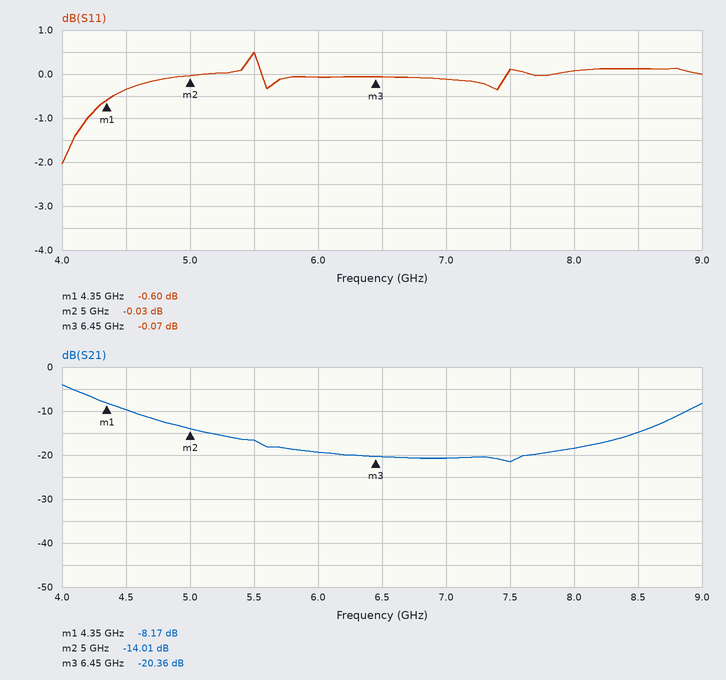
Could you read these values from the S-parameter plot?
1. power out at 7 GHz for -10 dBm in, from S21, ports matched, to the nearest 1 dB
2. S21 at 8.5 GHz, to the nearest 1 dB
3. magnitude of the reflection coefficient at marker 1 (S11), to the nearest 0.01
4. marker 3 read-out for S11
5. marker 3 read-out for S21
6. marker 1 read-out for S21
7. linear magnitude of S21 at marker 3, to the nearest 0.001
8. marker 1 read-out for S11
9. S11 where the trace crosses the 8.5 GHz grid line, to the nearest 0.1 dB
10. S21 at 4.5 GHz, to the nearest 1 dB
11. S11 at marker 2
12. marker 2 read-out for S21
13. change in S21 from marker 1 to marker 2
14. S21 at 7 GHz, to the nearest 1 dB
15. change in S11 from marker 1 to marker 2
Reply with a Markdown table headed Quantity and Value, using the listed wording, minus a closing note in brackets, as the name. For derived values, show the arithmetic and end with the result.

| Quantity | Value |
|---|---|
| power out at 7 GHz for -10 dBm in, from S21, ports matched, to the nearest 1 dB | -10 dBm + (-21 dB) = -31 dBm |
| S21 at 8.5 GHz, to the nearest 1 dB | -15 dB |
| magnitude of the reflection coefficient at marker 1 (S11), to the nearest 0.01 | 10^(-0.6/20) ≈ 0.93 |
| marker 3 read-out for S11 | -0.07 dB |
| marker 3 read-out for S21 | -20.36 dB |
| marker 1 read-out for S21 | -8.17 dB |
| linear magnitude of S21 at marker 3, to the nearest 0.001 | 10^(-20.36/20) ≈ 0.096 |
| marker 1 read-out for S11 | -0.60 dB |
| S11 where the trace crosses the 8.5 GHz grid line, to the nearest 0.1 dB | 0.1 dB |
| S21 at 4.5 GHz, to the nearest 1 dB | -10 dB |
| S11 at marker 2 | -0.03 dB |
| marker 2 read-out for S21 | -14.01 dB |
| change in S21 from marker 1 to marker 2 | -14.01 − (-8.17) = -5.84 dB |
| S21 at 7 GHz, to the nearest 1 dB | -21 dB |
| change in S11 from marker 1 to marker 2 | -0.03 − (-0.6) = 0.57 dB |
